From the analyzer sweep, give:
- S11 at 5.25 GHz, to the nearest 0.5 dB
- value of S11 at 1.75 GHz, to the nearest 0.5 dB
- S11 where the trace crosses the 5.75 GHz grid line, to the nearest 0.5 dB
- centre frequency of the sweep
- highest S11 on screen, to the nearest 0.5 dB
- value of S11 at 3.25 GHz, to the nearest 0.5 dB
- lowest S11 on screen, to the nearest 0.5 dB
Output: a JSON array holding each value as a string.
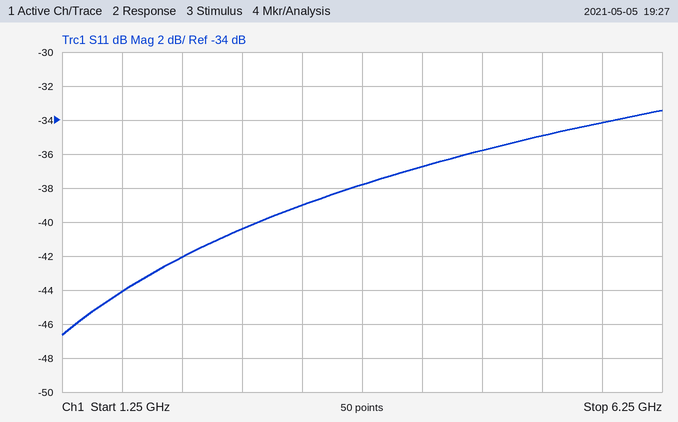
["-35.0 dB", "-44.0 dB", "-34.0 dB", "3.75 GHz", "-33.5 dB", "-39.0 dB", "-46.5 dB"]
